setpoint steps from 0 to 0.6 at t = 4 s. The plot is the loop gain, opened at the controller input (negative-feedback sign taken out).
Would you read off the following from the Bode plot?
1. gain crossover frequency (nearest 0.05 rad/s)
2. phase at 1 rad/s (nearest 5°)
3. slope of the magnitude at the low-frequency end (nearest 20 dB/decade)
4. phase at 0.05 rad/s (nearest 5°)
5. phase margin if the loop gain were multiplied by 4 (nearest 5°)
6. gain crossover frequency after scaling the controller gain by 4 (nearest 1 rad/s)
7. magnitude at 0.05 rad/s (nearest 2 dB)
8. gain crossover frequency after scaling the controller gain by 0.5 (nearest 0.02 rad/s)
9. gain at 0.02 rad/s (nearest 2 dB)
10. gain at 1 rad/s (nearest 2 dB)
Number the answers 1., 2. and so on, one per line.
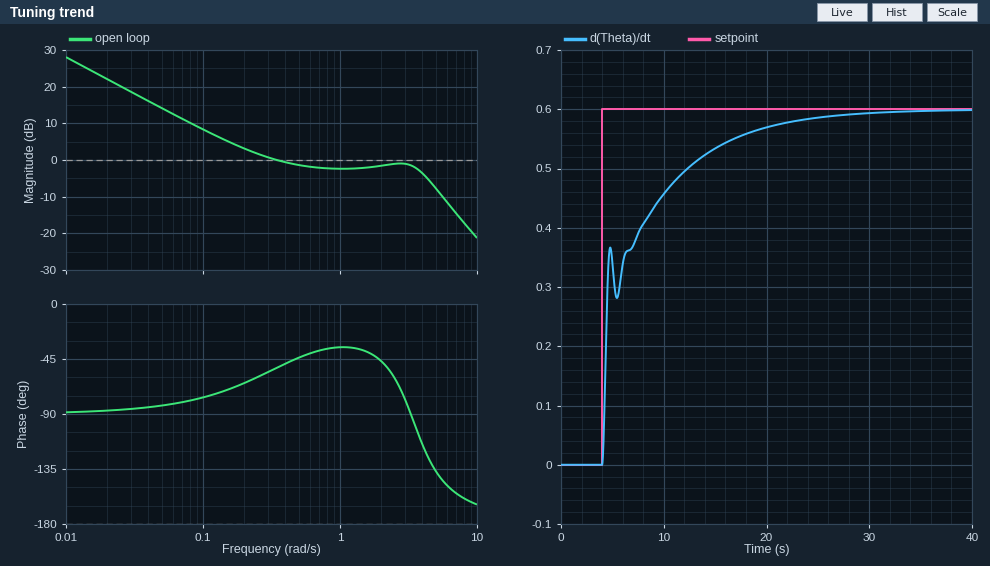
1. 0.35 rad/s
2. -35°
3. -20 dB/decade
4. -85°
5. 30°
6. 6 rad/s
7. 14 dB
8. 0.14 rad/s
9. 22 dB
10. -2 dB
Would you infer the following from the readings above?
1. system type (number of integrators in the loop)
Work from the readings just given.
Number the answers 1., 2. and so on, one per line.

1. 1
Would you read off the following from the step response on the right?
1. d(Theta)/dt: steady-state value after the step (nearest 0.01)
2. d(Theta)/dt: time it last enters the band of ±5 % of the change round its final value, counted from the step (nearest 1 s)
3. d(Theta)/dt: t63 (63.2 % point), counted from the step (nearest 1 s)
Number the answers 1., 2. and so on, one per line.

1. 0.60
2. 16 s
3. 3 s
